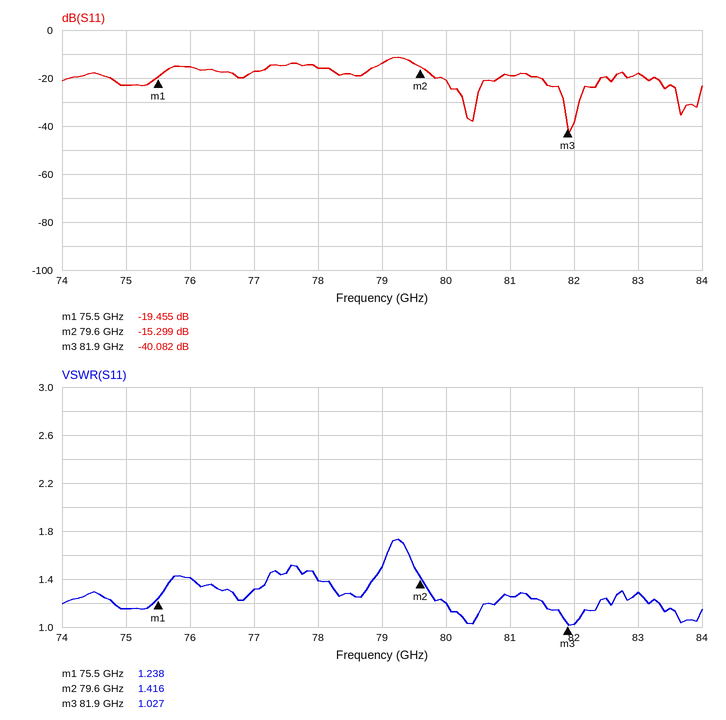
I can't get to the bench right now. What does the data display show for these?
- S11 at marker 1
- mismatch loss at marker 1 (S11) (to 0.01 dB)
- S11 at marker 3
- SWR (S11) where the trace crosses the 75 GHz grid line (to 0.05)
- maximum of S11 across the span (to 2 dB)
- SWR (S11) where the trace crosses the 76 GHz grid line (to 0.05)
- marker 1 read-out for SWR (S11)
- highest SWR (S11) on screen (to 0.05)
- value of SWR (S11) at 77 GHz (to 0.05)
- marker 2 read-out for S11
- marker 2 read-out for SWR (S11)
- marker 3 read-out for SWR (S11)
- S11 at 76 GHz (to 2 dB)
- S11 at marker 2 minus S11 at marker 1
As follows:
-19.455 dB
0.05 dB
-40.082 dB
1.15
-12 dB
1.40
1.238
1.75
1.30
-15.299 dB
1.416
1.027
-16 dB
4.156 dB
